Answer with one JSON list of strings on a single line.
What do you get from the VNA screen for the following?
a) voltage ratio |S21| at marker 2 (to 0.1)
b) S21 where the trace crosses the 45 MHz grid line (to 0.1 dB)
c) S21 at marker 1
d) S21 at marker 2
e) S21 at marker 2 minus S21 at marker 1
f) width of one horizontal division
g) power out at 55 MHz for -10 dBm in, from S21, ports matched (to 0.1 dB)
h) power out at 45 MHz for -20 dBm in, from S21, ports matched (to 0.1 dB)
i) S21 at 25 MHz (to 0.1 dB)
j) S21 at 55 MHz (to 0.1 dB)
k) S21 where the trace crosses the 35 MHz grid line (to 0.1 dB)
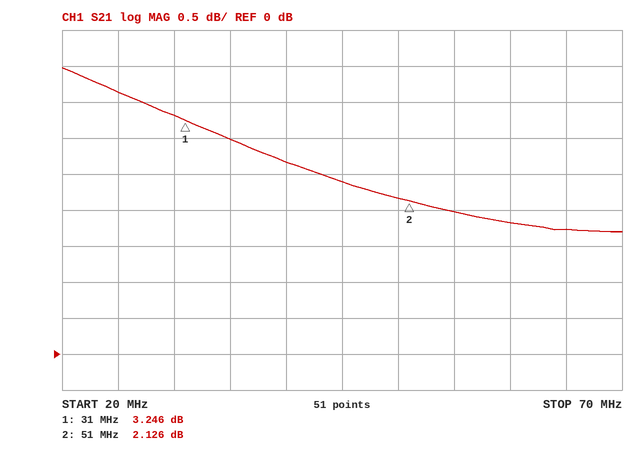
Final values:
["1.3", "2.4 dB", "3.246 dB", "2.126 dB", "-1.120 dB", "5 MHz", "-8.0 dBm", "-17.6 dBm", "3.6 dB", "2.0 dB", "3.0 dB"]
